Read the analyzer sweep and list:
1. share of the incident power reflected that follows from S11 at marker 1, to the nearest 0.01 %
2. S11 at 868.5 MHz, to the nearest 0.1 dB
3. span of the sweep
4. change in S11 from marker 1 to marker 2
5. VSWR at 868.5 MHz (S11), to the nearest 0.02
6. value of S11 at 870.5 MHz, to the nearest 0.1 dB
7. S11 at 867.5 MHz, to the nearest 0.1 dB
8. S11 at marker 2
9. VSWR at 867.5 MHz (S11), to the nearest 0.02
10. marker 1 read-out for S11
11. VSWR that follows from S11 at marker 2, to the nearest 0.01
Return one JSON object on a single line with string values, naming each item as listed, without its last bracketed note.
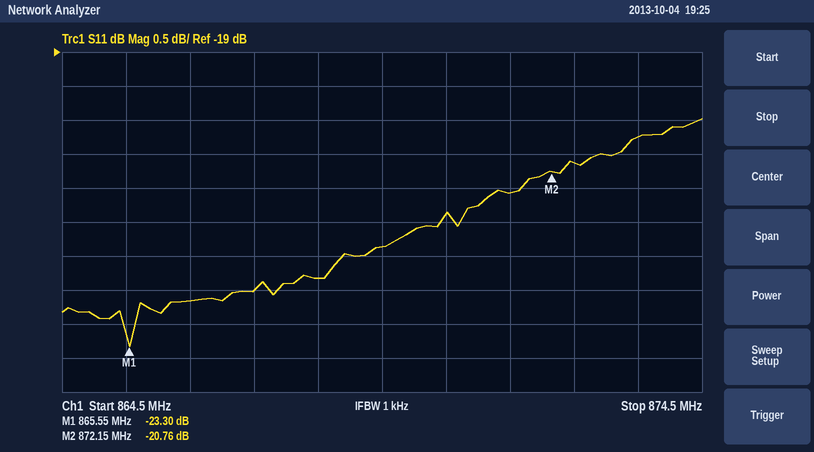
{"share of the incident power reflected that follows from S11 at marker 1, to the nearest 0.01 %": "0.47 %", "S11 at 868.5 MHz, to the nearest 0.1 dB": "-22.3 dB", "span of the sweep": "10 MHz", "change in S11 from marker 1 to marker 2": "2.54 dB", "VSWR at 868.5 MHz (S11), to the nearest 0.02": "1.16", "value of S11 at 870.5 MHz, to the nearest 0.1 dB": "-21.4 dB", "S11 at 867.5 MHz, to the nearest 0.1 dB": "-22.5 dB", "S11 at marker 2": "-20.76 dB", "VSWR at 867.5 MHz (S11), to the nearest 0.02": "1.16", "marker 1 read-out for S11": "-23.30 dB", "VSWR that follows from S11 at marker 2, to the nearest 0.01": "1.20"}
